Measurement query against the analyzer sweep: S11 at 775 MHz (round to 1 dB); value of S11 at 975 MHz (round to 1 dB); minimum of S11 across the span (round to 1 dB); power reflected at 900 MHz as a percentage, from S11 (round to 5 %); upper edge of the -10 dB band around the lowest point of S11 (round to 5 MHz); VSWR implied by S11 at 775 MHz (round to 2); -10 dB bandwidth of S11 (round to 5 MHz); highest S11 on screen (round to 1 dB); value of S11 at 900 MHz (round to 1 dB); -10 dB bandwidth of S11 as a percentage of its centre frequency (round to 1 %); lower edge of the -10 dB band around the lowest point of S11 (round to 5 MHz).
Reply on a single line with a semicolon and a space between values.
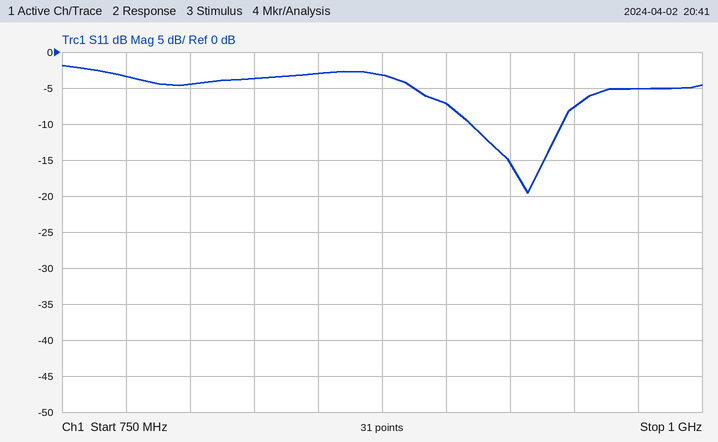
-3 dB; -5 dB; -20 dB; 20 %; 945 MHz; 6; 35 MHz; -2 dB; -7 dB; 4 %; 910 MHz
